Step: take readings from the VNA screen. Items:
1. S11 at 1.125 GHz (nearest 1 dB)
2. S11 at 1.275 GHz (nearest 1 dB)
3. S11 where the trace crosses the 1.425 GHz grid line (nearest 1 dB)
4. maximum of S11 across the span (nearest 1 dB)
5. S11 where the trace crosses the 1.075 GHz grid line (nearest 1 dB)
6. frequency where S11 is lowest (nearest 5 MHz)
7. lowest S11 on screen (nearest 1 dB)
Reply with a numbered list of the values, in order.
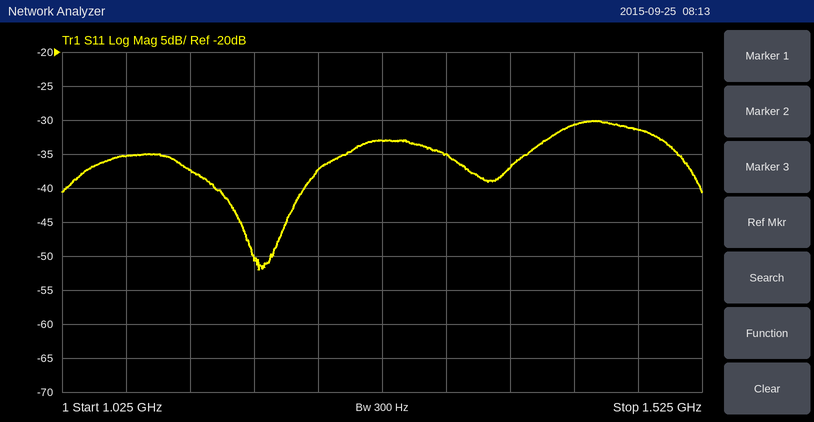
1. -37 dB
2. -33 dB
3. -31 dB
4. -30 dB
5. -35 dB
6. 1.180 GHz
7. -52 dB
